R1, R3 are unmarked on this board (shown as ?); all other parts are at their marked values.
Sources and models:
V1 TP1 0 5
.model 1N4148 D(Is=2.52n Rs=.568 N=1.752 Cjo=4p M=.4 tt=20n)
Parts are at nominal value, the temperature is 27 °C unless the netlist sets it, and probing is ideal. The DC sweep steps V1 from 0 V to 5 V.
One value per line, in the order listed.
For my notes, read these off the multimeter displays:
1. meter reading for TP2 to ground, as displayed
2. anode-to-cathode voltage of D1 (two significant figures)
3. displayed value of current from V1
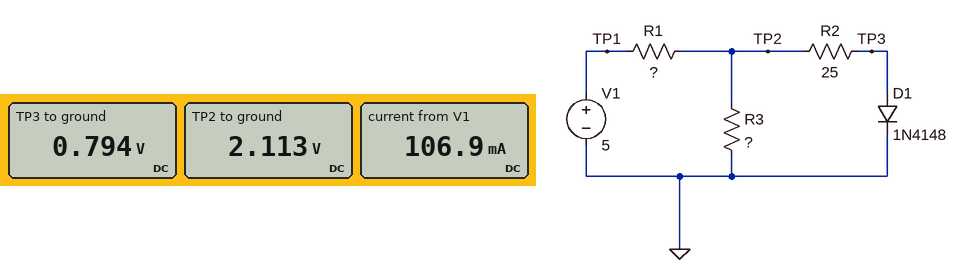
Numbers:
2.113 V
790 mV
106.9 mA
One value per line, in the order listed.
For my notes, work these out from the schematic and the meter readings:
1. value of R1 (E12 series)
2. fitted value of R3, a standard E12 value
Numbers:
27 Ω
39 Ω
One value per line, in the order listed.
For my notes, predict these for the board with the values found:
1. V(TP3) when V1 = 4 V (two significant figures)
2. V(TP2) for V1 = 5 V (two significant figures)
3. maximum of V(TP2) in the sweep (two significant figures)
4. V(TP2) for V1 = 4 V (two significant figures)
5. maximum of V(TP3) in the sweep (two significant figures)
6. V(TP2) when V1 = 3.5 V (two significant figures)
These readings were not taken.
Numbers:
770 mV
2.1 V
2.1 V
1.7 V
790 mV
1.6 V
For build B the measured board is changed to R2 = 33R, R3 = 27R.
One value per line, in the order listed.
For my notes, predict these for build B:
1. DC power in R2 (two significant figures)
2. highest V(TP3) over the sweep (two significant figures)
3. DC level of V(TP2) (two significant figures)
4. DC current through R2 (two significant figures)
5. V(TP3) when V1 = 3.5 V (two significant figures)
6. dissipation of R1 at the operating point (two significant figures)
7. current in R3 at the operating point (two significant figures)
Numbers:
46 mW
770 mV
2.0 V
37 mA
740 mV
330 mW
74 mA
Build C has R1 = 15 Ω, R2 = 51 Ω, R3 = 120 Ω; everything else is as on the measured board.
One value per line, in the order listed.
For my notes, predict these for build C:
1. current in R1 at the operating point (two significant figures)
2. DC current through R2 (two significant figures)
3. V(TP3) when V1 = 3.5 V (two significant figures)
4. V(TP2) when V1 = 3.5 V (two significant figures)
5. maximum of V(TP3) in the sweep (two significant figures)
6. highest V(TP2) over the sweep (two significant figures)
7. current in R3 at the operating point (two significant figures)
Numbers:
87 mA
57 mA
770 mV
2.6 V
800 mV
3.7 V
31 mA
